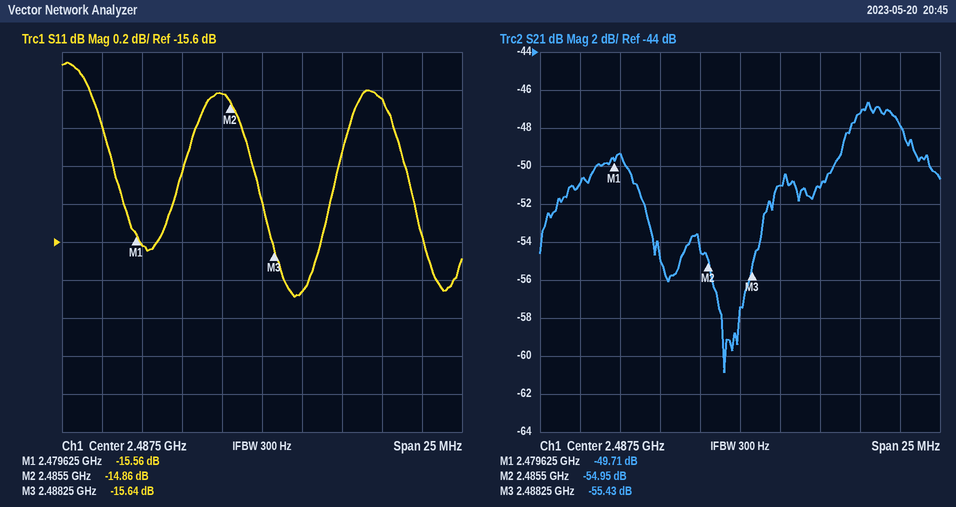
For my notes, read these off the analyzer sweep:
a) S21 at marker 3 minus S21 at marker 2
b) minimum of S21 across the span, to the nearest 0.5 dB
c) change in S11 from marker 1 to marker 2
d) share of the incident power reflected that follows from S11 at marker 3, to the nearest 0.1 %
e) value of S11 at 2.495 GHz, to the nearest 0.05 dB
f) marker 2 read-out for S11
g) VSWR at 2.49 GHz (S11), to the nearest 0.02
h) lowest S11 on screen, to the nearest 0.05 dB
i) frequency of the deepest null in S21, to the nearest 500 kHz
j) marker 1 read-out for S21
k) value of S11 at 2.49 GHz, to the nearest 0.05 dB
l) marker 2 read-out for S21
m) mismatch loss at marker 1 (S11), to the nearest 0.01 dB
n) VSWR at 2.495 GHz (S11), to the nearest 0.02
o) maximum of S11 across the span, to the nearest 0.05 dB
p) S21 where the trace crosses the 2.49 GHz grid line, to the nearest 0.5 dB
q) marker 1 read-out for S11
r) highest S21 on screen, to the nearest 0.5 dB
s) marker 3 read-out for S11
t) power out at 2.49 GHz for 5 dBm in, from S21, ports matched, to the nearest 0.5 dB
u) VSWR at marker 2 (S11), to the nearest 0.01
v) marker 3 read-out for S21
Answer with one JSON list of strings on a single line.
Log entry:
["-0.48 dB", "-61.0 dB", "0.70 dB", "2.7 %", "-14.85 dB", "-14.86 dB", "1.38", "-15.90 dB", "2.4865 GHz", "-49.71 dB", "-15.85 dB", "-54.95 dB", "0.12 dB", "1.44", "-14.65 dB", "-51.0 dB", "-15.56 dB", "-46.5 dB", "-15.64 dB", "-46.0 dBm", "1.44", "-55.43 dB"]
